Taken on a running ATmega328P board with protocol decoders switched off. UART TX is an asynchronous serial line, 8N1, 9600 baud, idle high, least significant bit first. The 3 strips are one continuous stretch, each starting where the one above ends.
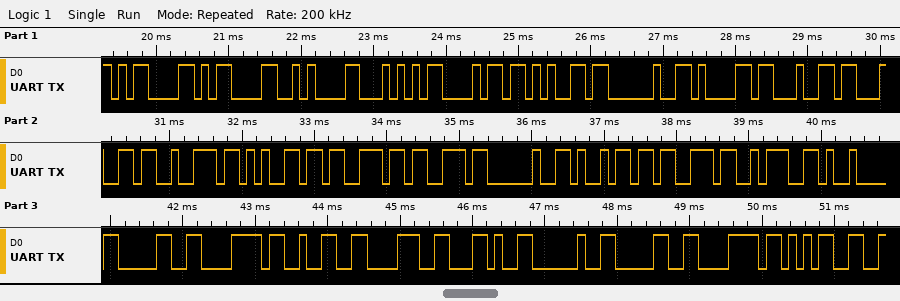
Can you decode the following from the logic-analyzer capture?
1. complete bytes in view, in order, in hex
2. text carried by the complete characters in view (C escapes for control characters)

0x0D 0x0D 0x0A 0x54 0x68 0x65 0x20 0x61 0x64 0x64 0x72 0x65 0x73 0x73 0x20 0x69 0x73 0x3A 0x09 0x30 0x78 0x32 0x38 0x2C 0x20 0x30 0x78 0x35
"\r\r\nThe address is:\t0x28, 0x5"
